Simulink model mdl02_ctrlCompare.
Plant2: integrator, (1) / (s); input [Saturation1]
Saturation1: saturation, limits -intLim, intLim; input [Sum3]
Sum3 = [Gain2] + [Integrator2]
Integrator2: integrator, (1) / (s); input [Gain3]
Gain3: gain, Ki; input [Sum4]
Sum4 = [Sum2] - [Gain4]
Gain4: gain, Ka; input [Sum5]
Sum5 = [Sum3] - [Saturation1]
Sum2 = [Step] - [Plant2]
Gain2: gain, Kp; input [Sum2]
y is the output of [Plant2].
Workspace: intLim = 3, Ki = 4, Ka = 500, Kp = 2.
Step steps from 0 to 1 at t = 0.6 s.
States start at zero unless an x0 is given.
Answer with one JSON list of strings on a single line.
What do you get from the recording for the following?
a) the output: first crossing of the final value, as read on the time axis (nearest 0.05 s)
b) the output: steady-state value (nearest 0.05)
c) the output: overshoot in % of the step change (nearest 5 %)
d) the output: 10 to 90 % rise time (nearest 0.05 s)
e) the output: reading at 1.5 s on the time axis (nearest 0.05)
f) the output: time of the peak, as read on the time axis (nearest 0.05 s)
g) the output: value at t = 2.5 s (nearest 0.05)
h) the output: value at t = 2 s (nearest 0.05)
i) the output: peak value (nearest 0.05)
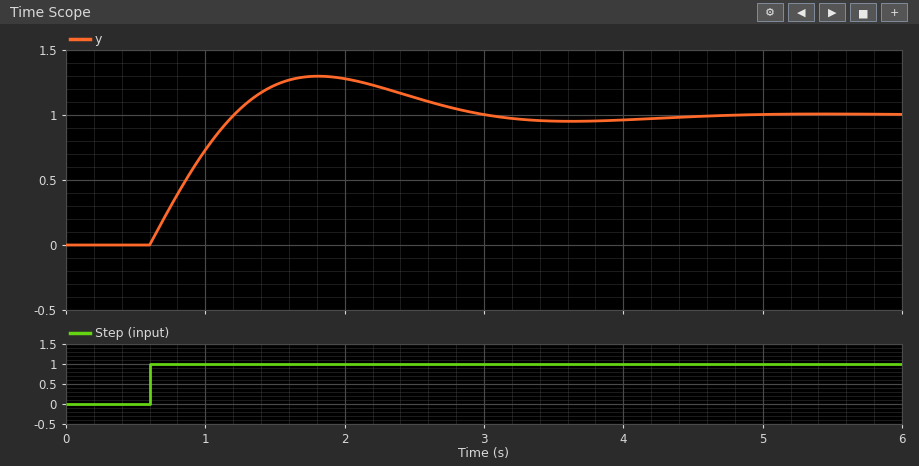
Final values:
["1.20 s", "1.00", "30 %", "0.45 s", "1.25", "1.80 s", "1.15", "1.30", "1.30"]
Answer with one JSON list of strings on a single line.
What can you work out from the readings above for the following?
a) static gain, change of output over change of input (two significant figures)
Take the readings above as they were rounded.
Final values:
["1.0"]
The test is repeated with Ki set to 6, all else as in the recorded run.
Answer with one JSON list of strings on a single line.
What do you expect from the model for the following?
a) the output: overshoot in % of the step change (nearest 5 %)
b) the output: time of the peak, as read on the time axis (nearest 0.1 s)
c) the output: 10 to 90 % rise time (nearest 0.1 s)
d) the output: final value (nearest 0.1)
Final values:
["35 %", "1.6 s", "0.4 s", "1.0"]
